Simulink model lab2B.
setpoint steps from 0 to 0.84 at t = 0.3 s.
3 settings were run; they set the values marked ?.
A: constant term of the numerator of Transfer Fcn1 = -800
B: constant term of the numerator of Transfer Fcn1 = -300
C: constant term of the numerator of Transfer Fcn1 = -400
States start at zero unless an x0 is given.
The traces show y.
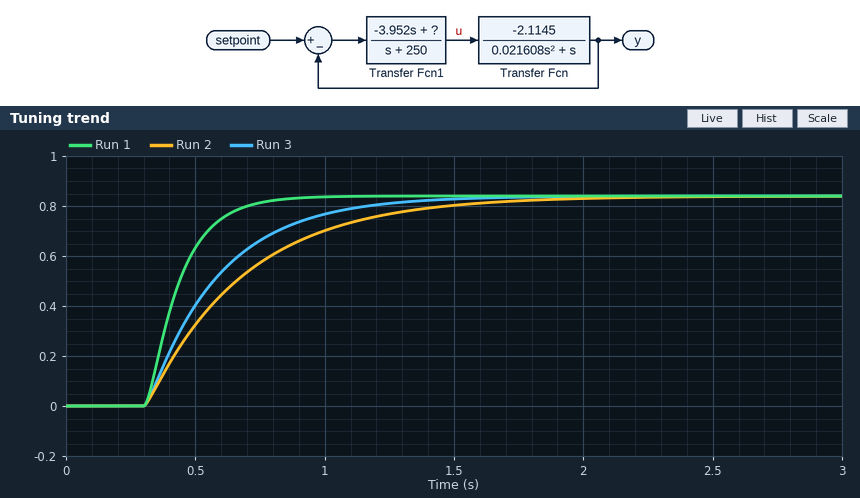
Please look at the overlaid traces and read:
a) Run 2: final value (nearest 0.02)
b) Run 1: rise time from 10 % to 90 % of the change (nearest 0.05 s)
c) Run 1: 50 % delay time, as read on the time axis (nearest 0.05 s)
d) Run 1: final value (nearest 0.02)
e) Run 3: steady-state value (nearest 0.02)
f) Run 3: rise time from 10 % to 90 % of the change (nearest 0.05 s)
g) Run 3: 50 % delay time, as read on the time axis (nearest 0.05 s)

0.84
0.30 s
0.40 s
0.84
0.84
0.60 s
0.50 s
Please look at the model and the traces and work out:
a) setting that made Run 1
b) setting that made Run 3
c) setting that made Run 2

A
C
B
